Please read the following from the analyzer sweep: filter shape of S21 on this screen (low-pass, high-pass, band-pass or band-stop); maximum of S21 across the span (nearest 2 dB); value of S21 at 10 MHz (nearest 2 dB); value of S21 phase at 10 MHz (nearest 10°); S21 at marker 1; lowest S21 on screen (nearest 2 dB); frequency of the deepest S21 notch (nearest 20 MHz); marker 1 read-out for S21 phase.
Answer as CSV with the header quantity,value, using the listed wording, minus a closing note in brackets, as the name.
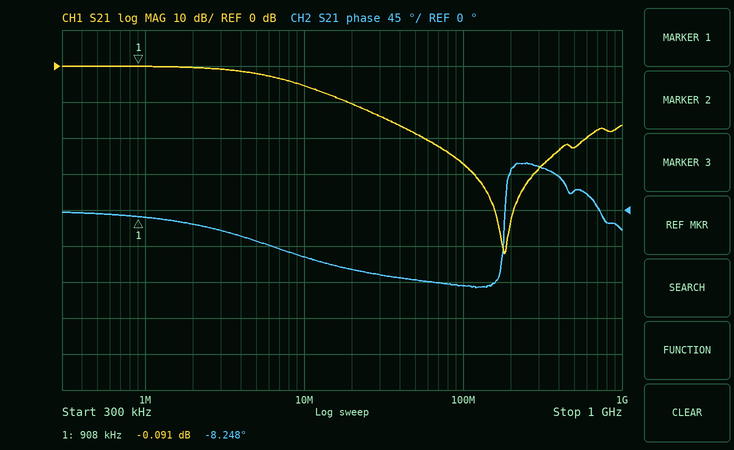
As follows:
quantity,value
filter shape of S21 on this screen,low-pass
maximum of S21 across the span,0 dB
value of S21 at 10 MHz,-6 dB
value of S21 phase at 10 MHz,-60°
S21 at marker 1,-0.091 dB
lowest S21 on screen,-52 dB
frequency of the deepest S21 notch,180 MHz
marker 1 read-out for S21 phase,-8.248°
